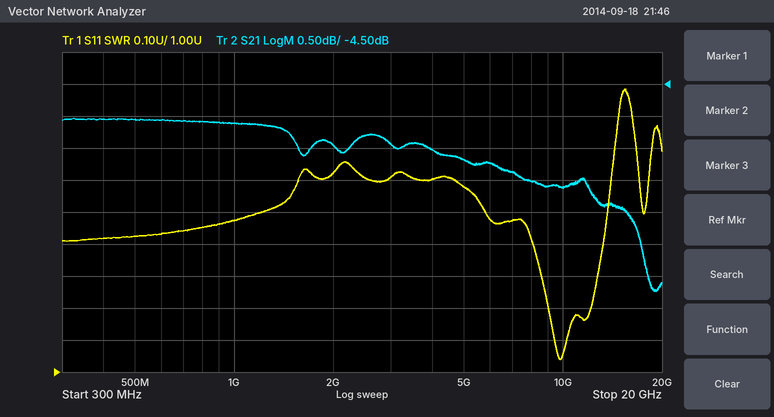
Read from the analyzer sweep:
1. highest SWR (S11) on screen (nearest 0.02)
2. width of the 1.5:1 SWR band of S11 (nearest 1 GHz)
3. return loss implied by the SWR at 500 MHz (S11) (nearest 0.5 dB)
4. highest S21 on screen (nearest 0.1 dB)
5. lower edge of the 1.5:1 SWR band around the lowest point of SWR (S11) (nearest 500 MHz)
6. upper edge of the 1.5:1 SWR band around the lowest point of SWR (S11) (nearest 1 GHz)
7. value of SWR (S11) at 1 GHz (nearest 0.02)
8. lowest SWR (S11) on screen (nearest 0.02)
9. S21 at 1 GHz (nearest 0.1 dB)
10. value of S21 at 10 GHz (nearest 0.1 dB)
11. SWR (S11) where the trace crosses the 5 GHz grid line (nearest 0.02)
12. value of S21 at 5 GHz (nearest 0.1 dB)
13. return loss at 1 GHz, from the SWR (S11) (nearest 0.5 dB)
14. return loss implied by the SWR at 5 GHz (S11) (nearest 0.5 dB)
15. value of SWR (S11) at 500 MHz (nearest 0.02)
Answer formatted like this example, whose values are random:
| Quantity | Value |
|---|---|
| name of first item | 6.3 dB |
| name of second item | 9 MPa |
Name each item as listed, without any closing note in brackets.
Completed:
| Quantity | Value |
|---|---|
| highest SWR (S11) on screen | 1.88 |
| width of the 1.5:1 SWR band of S11 | 8 GHz |
| return loss implied by the SWR at 500 MHz (S11) | 15.0 dB |
| highest S21 on screen | -5.0 dB |
| lower edge of the 1.5:1 SWR band around the lowest point of SWR (S11) | 6.0 GHz |
| upper edge of the 1.5:1 SWR band around the lowest point of SWR (S11) | 14 GHz |
| value of SWR (S11) at 1 GHz | 1.48 |
| lowest SWR (S11) on screen | 1.04 |
| S21 at 1 GHz | -5.1 dB |
| value of S21 at 10 GHz | -6.1 dB |
| SWR (S11) where the trace crosses the 5 GHz grid line | 1.58 |
| value of S21 at 5 GHz | -5.7 dB |
| return loss at 1 GHz, from the SWR (S11) | 14.5 dB |
| return loss implied by the SWR at 5 GHz (S11) | 13.0 dB |
| value of SWR (S11) at 500 MHz | 1.42 |
